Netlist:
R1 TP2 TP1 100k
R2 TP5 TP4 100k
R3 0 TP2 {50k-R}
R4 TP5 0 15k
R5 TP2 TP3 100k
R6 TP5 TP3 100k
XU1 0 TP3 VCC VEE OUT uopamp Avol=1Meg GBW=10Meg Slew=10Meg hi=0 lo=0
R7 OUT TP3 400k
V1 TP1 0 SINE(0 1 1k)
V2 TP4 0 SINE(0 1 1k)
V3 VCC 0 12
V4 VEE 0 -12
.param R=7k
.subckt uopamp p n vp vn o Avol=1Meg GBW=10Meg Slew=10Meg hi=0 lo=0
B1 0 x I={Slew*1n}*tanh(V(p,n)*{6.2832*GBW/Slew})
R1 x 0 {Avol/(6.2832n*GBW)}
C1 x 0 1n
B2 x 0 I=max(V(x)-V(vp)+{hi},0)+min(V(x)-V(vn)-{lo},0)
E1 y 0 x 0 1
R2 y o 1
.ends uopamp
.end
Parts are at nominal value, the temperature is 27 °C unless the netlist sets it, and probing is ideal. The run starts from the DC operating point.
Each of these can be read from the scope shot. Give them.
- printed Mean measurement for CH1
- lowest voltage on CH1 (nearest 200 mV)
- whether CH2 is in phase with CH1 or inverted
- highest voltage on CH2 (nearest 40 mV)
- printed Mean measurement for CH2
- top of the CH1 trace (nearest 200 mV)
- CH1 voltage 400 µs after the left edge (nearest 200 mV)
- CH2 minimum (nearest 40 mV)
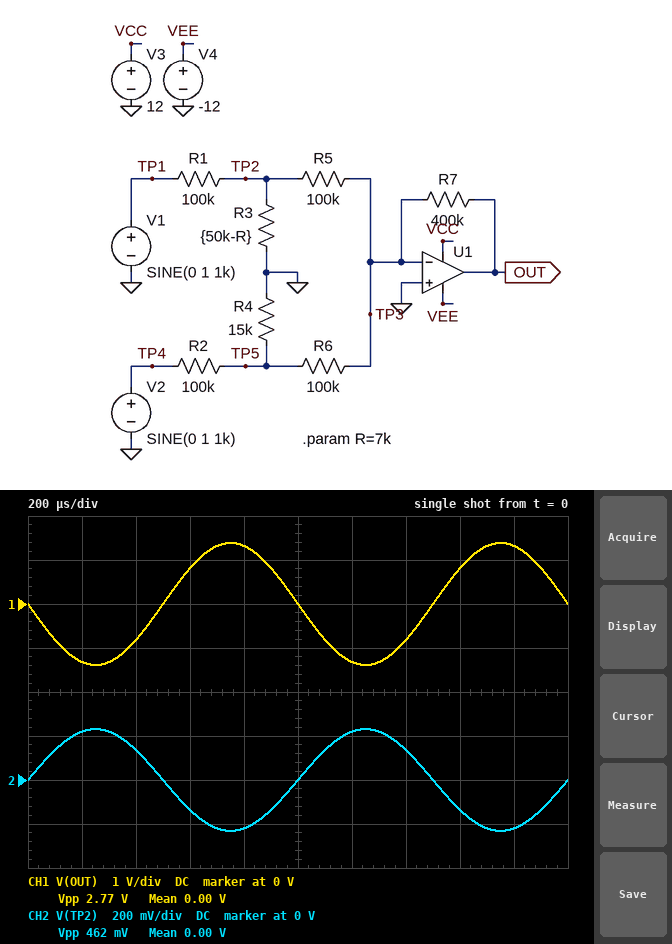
0.00 V
-1.4 V
inverted
240 mV
0.00 V
1.4 V
-800 mV
-240 mV
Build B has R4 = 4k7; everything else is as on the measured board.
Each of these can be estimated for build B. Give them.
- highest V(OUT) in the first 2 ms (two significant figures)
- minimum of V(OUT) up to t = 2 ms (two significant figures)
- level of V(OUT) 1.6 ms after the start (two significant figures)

1.1 V
-1.1 V
640 mV
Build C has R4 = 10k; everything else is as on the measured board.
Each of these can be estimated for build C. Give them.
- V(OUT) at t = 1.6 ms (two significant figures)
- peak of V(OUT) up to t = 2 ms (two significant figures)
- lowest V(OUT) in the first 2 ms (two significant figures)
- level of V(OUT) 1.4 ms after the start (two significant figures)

740 mV
1.3 V
-1.3 V
-740 mV
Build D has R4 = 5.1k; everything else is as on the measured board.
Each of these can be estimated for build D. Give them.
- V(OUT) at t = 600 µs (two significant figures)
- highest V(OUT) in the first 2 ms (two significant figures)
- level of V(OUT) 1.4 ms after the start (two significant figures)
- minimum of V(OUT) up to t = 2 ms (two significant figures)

650 mV
1.1 V
-650 mV
-1.1 V
